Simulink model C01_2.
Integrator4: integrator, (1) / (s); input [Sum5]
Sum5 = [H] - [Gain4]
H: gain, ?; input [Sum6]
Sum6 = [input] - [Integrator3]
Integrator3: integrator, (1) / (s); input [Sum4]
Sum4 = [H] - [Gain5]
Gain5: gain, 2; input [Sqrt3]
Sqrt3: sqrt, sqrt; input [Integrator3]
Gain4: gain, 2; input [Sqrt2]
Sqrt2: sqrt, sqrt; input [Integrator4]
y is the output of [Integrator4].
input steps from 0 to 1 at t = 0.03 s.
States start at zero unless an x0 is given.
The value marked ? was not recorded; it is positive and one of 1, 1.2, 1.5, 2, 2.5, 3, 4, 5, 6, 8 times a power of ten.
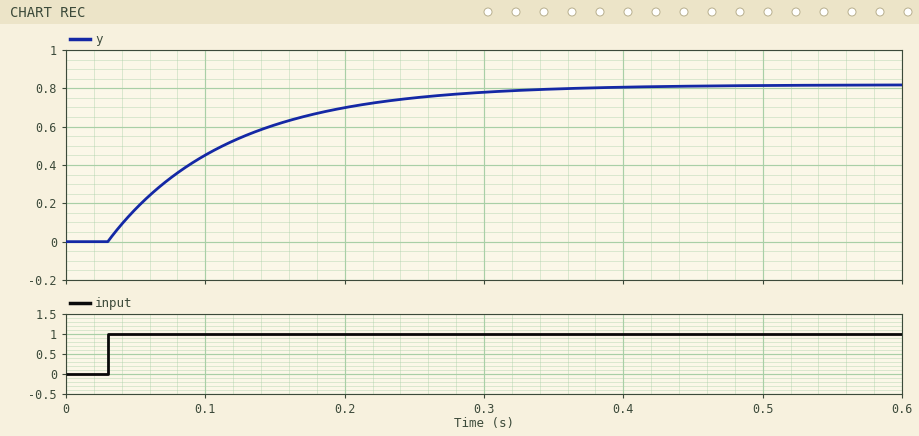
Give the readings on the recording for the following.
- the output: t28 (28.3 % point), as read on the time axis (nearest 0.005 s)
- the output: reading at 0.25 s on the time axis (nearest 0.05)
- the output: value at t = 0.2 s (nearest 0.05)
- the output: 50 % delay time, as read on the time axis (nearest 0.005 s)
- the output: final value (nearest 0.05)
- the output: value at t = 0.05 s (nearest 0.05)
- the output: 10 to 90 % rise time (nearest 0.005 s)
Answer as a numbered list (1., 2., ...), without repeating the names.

1. 0.060 s
2. 0.75
3. 0.70
4. 0.090 s
5. 0.80
6. 0.15
7. 0.195 s
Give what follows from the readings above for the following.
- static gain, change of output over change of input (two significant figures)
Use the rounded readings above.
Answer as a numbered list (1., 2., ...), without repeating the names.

1. 0.80
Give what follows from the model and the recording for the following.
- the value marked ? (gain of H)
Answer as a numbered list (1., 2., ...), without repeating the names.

1. 10
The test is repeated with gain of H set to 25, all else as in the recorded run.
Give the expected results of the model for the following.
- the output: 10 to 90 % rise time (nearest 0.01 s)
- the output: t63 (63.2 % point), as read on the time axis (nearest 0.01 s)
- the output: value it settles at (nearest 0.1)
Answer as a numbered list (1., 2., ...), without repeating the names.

1. 0.08 s
2. 0.07 s
3. 0.9
